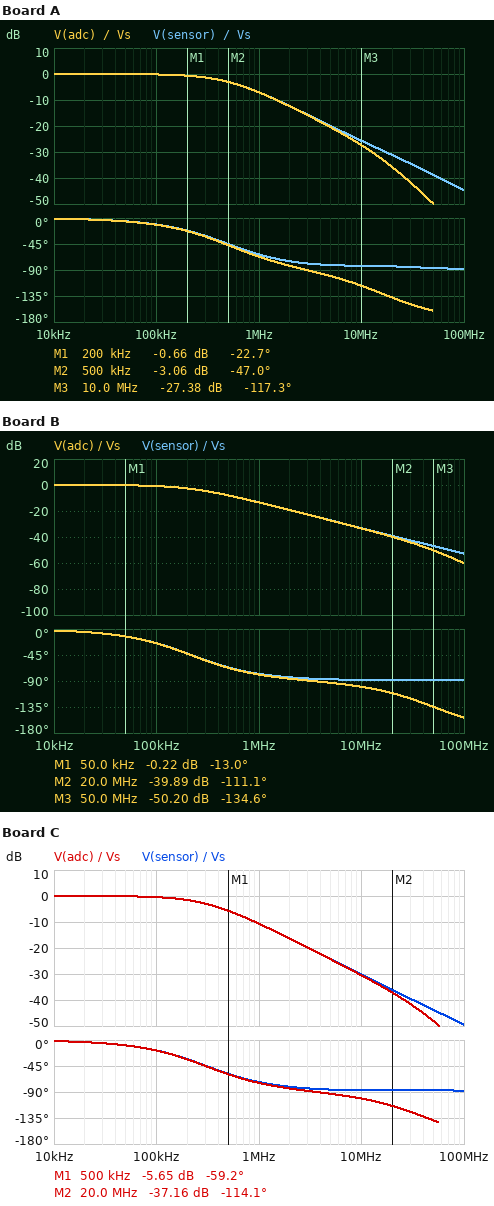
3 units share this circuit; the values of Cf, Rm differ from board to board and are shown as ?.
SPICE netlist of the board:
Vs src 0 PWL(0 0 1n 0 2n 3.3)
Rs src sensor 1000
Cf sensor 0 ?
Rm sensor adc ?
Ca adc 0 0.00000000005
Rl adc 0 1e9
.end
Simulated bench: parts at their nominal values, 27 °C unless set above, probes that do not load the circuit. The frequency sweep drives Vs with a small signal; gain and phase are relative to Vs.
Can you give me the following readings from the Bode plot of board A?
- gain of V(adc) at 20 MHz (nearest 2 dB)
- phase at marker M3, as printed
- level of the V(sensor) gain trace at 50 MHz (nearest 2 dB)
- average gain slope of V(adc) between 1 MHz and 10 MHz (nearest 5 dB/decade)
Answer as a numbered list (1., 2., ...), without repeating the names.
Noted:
1. -36 dB
2. -117.3 deg
3. -38 dB
4. -20 dB/decade
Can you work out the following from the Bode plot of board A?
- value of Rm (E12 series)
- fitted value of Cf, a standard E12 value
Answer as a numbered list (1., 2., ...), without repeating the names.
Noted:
1. 220 Ω
2. 270 pF
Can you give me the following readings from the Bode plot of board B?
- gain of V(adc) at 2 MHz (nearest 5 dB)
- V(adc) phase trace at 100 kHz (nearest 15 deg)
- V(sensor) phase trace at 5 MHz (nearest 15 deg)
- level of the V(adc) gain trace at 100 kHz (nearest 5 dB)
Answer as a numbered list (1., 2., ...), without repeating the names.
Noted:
1. -20 dB
2. -30 deg
3. -90 deg
4. 0 dB
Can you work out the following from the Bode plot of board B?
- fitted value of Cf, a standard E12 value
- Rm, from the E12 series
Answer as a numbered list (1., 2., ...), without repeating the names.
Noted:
1. 680 pF
2. 68 Ω
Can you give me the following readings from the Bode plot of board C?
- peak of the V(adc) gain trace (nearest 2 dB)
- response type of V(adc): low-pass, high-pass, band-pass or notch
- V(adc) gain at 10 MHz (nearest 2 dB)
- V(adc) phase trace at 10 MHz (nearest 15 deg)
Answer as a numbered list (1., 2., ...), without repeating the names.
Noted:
1. 0 dB
2. low-pass
3. -30 dB
4. -105 deg
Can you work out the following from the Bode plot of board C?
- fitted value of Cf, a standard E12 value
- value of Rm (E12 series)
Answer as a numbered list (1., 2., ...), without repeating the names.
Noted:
1. 470 pF
2. 82 Ω
